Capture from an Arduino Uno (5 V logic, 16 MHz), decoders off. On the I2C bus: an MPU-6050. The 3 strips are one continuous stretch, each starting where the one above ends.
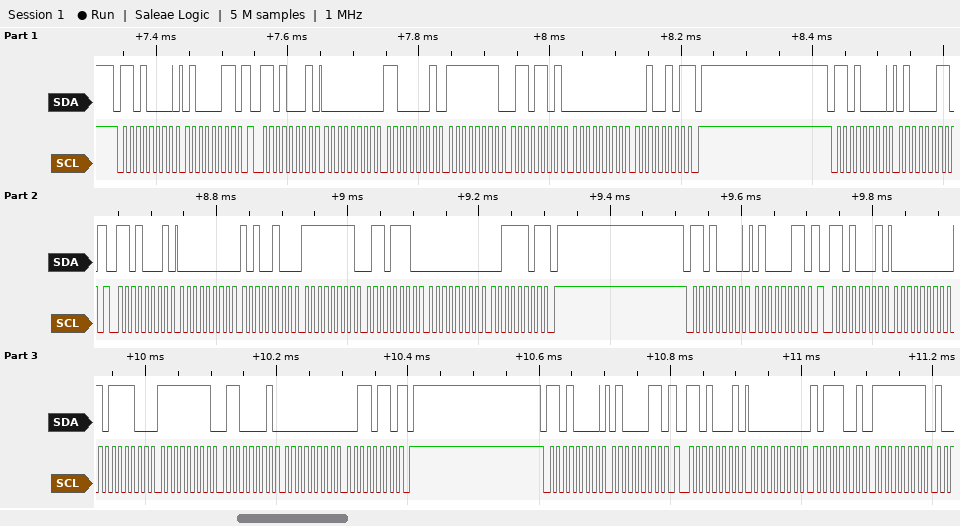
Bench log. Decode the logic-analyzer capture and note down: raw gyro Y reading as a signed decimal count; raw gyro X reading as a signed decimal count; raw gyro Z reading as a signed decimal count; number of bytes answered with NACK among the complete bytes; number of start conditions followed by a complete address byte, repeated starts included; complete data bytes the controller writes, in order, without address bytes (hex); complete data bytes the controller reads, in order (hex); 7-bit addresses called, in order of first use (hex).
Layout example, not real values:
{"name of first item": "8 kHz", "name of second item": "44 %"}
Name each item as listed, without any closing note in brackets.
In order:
{"raw gyro Y reading as a signed decimal count": "-147", "raw gyro X reading as a signed decimal count": "193", "raw gyro Z reading as a signed decimal count": "37", "number of bytes answered with NACK among the complete bytes": "3", "number of start conditions followed by a complete address byte, repeated starts included": "8", "complete data bytes the controller writes, in order, without address bytes": "43 43 43 43", "complete data bytes the controller reads, in order": "00 C1 FF 6D 00 25 00 A4 FF 6E 00 3D 00 BC FF 61 00 36 00 B9 FF", "7-bit addresses called, in order of first use": "0x68"}
